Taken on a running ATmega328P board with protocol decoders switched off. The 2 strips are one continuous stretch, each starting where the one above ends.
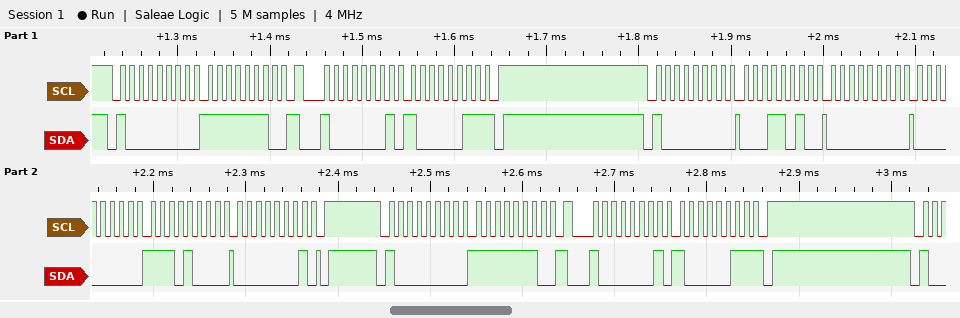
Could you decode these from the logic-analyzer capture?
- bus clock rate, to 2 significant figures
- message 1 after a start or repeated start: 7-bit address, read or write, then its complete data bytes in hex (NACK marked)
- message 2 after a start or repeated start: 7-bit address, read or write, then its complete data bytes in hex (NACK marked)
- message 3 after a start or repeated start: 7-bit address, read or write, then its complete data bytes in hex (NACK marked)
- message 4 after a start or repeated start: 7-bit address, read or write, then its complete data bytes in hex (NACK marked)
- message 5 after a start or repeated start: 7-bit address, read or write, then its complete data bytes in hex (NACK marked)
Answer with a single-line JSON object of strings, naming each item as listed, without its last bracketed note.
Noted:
{"bus clock rate, to 2 significant figures": "100 kHz", "message 1 after a start or repeated start: 7-bit address, read or write, then its complete data bytes in hex": "0x40 write: FE", "message 2 after a start or repeated start: 7-bit address, read or write, then its complete data bytes in hex": "0x40 read: 83 NACK", "message 3 after a start or repeated start: 7-bit address, read or write, then its complete data bytes in hex": "0x40 write: 1A 00 00 E8 01", "message 4 after a start or repeated start: 7-bit address, read or write, then its complete data bytes in hex": "0x40 write: FE", "message 5 after a start or repeated start: 7-bit address, read or write, then its complete data bytes in hex": "0x40 read: 83 NACK"}
